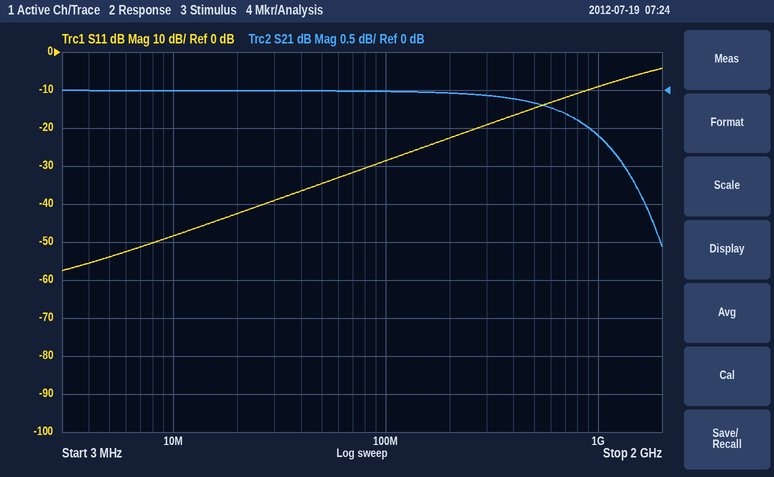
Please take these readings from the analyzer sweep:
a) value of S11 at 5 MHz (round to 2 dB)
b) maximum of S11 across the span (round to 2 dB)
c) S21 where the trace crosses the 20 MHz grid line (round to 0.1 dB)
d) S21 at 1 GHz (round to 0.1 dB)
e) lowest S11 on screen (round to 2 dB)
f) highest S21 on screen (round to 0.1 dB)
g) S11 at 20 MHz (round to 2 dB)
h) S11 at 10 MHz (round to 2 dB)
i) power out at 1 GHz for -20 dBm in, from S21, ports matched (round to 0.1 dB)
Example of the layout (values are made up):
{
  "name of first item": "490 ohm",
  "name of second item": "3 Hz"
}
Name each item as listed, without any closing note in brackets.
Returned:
{
  "value of S11 at 5 MHz": "-54 dB",
  "maximum of S11 across the span": "-4 dB",
  "S21 where the trace crosses the 20 MHz grid line": "0.0 dB",
  "S21 at 1 GHz": "-0.6 dB",
  "lowest S11 on screen": "-58 dB",
  "highest S21 on screen": "0.0 dB",
  "S11 at 20 MHz": "-42 dB",
  "S11 at 10 MHz": "-48 dB",
  "power out at 1 GHz for -20 dBm in, from S21, ports matched": "-20.6 dBm"
}
